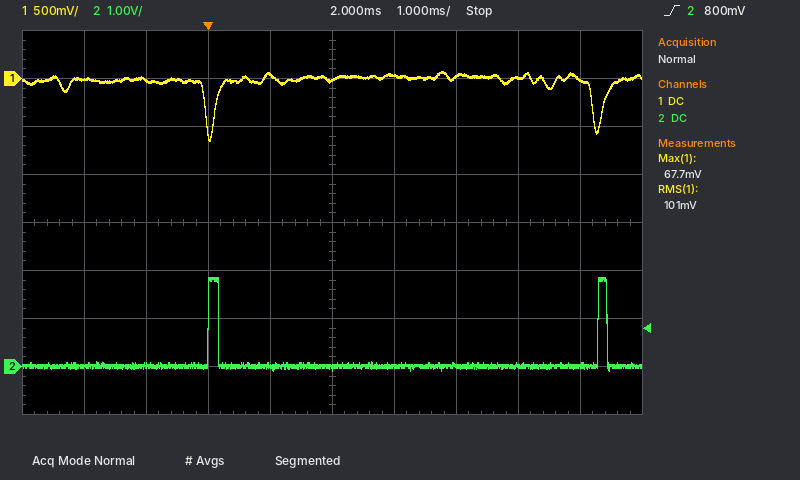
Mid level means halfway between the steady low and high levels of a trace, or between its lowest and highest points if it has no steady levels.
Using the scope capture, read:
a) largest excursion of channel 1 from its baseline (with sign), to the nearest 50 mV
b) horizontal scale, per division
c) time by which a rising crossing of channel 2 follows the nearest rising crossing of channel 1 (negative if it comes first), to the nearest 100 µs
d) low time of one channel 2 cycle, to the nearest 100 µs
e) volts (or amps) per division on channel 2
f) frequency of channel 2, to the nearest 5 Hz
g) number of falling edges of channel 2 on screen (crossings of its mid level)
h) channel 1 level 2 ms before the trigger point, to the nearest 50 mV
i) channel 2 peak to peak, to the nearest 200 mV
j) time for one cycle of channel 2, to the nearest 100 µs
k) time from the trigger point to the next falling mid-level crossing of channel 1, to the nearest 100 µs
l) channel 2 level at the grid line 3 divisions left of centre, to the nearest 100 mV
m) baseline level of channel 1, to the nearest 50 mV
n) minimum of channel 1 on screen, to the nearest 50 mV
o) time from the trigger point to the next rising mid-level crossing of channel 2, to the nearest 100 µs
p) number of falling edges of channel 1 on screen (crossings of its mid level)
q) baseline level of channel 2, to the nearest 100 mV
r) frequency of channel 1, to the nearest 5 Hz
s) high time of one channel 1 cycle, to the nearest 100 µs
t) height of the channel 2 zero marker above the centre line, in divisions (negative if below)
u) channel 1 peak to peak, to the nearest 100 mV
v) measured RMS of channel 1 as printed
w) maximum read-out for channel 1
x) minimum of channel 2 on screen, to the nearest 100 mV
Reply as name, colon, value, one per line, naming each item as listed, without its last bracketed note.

largest excursion of channel 1 from its baseline (with sign), to the nearest 50 mV: -650 mV
horizontal scale, per division: 1 ms
time by which a rising crossing of channel 2 follows the nearest rising crossing of channel 1 (negative if it comes first), to the nearest 100 µs: -100 µs
low time of one channel 2 cycle, to the nearest 100 µs: 6.1 ms
volts (or amps) per division on channel 2: 1 V
frequency of channel 2, to the nearest 5 Hz: 160 Hz
number of falling edges of channel 2 on screen: 2
channel 1 level 2 ms before the trigger point, to the nearest 50 mV: 0 mV
channel 2 peak to peak, to the nearest 200 mV: 2.0 V
time for one cycle of channel 2, to the nearest 100 µs: 6.3 ms
time from the trigger point to the next falling mid-level crossing of channel 1, to the nearest 100 µs: 6.2 ms
channel 2 level at the grid line 3 divisions left of centre, to the nearest 100 mV: 0.0 V
baseline level of channel 1, to the nearest 50 mV: 0 mV
minimum of channel 1 on screen, to the nearest 50 mV: -650 mV
time from the trigger point to the next rising mid-level crossing of channel 2, to the nearest 100 µs: 6.3 ms
number of falling edges of channel 1 on screen: 2
baseline level of channel 2, to the nearest 100 mV: 0.0 V
frequency of channel 1, to the nearest 5 Hz: 160 Hz
high time of one channel 1 cycle, to the nearest 100 µs: 6.1 ms
height of the channel 2 zero marker above the centre line, in divisions: -3.0 div
channel 1 peak to peak, to the nearest 100 mV: 700 mV
measured RMS of channel 1 as printed: 101 mV
maximum read-out for channel 1: 67.7 mV
minimum of channel 2 on screen, to the nearest 100 mV: -100 mV
